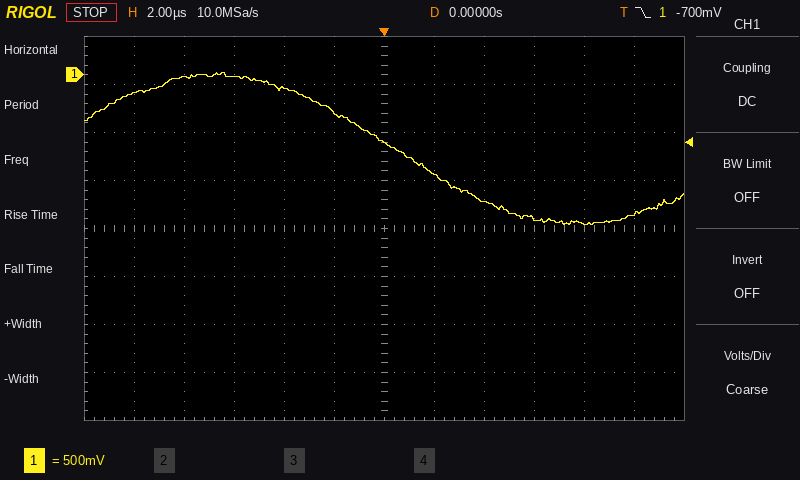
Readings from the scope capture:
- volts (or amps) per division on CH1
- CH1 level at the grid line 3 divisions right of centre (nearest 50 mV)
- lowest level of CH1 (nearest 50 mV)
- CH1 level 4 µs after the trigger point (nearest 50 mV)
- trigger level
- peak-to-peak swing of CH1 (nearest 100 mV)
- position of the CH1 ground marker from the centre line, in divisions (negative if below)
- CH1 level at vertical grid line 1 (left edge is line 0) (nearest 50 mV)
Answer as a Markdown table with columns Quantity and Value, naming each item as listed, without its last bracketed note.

| Quantity | Value |
|---|---|
| volts (or amps) per division on CH1 | 500 mV |
| CH1 level at the grid line 3 divisions right of centre | -1.50 V |
| lowest level of CH1 | -1.55 V |
| CH1 level 4 µs after the trigger point | -1.30 V |
| trigger level | -700 mV |
| peak-to-peak swing of CH1 | 1.60 V |
| position of the CH1 ground marker from the centre line, in divisions | +3.2 div |
| CH1 level at vertical grid line 1 (left edge is line 0) | -200 mV |
